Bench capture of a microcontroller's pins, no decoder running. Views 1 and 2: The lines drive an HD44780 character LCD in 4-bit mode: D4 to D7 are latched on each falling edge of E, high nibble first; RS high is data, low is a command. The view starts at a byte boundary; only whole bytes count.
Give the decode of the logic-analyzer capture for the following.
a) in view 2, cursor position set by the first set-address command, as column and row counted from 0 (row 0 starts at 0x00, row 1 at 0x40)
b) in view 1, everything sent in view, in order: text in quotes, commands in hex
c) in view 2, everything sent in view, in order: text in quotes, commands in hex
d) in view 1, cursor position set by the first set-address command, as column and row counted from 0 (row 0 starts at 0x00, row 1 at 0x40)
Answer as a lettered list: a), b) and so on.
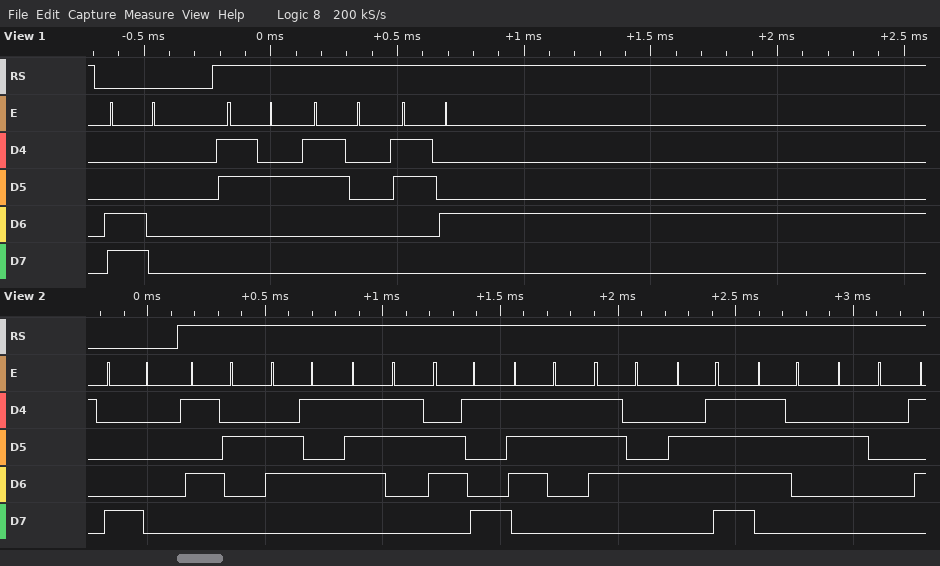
a) column 0, row 0
b) 0xC0 "204"
c) 0x80 "Resistor "
d) column 0, row 1
